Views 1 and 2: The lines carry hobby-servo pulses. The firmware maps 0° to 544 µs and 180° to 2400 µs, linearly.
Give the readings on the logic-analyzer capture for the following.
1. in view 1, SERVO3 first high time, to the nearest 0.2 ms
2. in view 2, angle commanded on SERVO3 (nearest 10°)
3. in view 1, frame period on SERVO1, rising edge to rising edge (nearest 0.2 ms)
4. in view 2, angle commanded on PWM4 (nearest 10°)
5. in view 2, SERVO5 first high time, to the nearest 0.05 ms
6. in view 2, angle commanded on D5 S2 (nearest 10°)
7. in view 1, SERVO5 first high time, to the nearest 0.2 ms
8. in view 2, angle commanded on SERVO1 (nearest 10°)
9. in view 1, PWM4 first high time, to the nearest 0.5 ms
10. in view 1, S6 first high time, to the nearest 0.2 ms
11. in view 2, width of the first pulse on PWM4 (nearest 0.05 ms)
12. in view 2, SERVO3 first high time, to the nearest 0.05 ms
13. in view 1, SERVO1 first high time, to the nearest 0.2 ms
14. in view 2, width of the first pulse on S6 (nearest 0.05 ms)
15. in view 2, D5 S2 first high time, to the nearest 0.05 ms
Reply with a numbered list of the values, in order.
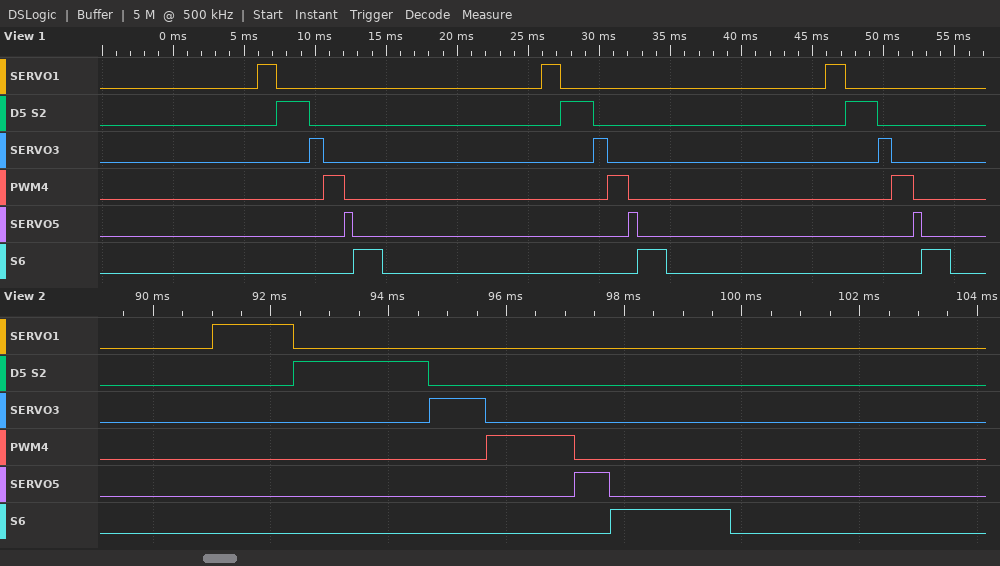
1. 1.0 ms
2. 40°
3. 20.0 ms
4. 90°
5. 0.60 ms
6. 170°
7. 0.6 ms
8. 80°
9. 1.5 ms
10. 2.0 ms
11. 1.50 ms
12. 0.95 ms
13. 1.4 ms
14. 2.05 ms
15. 2.30 ms
